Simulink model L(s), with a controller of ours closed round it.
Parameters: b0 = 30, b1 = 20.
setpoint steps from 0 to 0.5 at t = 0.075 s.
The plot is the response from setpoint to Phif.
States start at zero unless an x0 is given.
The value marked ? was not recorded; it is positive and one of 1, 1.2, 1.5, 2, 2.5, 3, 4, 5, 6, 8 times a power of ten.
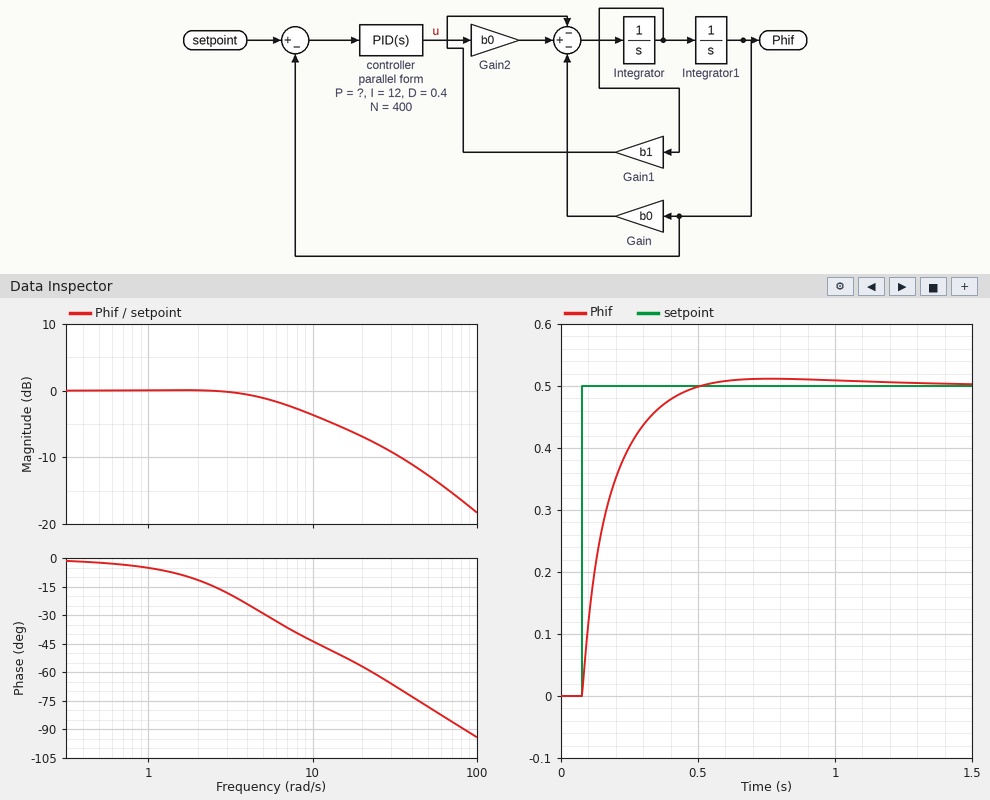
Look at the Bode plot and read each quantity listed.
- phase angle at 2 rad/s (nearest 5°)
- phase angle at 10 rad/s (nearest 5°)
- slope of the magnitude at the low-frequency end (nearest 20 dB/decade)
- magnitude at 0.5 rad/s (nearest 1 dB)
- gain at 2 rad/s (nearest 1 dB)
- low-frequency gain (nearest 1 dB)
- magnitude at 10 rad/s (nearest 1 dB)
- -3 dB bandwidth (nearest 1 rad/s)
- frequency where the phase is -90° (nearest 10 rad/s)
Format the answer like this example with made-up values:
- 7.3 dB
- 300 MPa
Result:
- -10°
- -45°
- 0 dB/decade
- 0 dB
- 0 dB
- 0 dB
- -4 dB
- 9 rad/s
- 80 rad/s
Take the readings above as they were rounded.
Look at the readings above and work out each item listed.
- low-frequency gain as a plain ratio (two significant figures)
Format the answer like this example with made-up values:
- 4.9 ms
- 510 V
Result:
- 1.0
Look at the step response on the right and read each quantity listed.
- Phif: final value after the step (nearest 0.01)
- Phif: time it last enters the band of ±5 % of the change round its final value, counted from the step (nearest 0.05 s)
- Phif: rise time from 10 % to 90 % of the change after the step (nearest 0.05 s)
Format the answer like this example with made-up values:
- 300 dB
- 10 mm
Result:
- 0.50
- 0.30 s
- 0.25 s
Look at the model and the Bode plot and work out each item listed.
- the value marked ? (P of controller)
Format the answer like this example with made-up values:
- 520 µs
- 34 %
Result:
- 6
